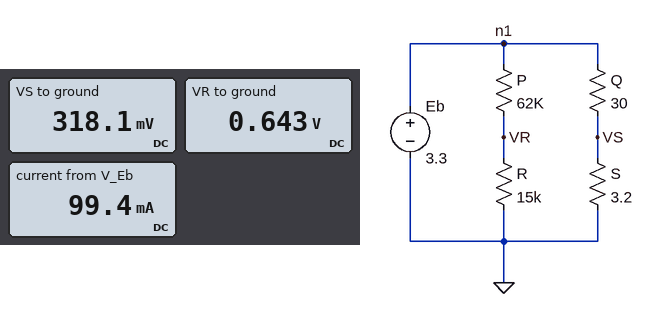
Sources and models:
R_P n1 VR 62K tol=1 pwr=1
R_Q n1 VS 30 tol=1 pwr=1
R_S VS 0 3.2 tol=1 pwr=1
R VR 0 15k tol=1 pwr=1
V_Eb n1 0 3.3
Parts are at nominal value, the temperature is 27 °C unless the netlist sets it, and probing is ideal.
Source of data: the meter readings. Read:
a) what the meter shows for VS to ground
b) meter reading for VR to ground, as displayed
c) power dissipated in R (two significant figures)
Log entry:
318.1 mV
0.643 V
28 µW
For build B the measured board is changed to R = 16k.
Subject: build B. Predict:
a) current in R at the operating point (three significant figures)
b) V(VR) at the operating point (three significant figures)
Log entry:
42.3 µA
677 mV
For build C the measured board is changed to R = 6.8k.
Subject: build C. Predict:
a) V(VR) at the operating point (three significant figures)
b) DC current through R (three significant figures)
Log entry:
326 mV
48.0 µA
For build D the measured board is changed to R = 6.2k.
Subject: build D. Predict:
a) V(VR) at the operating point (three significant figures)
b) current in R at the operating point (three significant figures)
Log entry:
300 mV
48.4 µA
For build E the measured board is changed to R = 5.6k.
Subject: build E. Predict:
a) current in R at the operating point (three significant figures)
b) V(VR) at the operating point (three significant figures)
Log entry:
48.8 µA
273 mV
